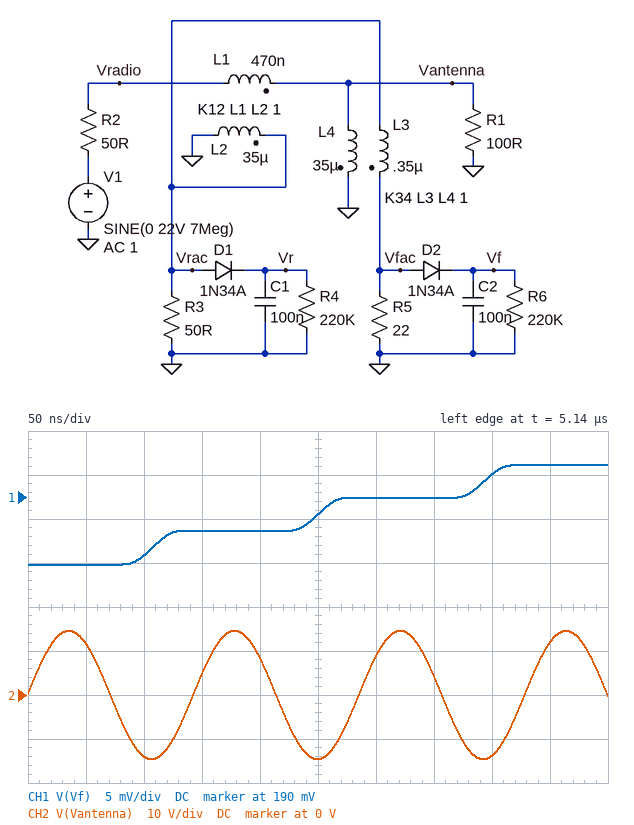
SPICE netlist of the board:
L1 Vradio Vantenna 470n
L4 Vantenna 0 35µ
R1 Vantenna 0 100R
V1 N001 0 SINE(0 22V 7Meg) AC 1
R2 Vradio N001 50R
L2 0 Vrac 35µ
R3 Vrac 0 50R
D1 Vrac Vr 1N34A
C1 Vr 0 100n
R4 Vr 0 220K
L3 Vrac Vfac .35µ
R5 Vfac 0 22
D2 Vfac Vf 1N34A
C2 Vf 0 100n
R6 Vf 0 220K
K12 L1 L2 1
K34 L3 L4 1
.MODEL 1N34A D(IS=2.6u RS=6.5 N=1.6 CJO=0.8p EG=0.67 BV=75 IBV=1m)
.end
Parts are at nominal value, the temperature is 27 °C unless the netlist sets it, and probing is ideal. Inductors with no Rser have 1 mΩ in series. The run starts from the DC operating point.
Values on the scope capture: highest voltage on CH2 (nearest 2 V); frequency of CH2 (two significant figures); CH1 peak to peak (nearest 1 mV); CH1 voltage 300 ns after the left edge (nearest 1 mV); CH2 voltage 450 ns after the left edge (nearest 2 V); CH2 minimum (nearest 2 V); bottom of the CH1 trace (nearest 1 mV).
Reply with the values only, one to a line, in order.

14 V
7.0 MHz
11 mV
190 mV
12 V
-14 V
182 mV
